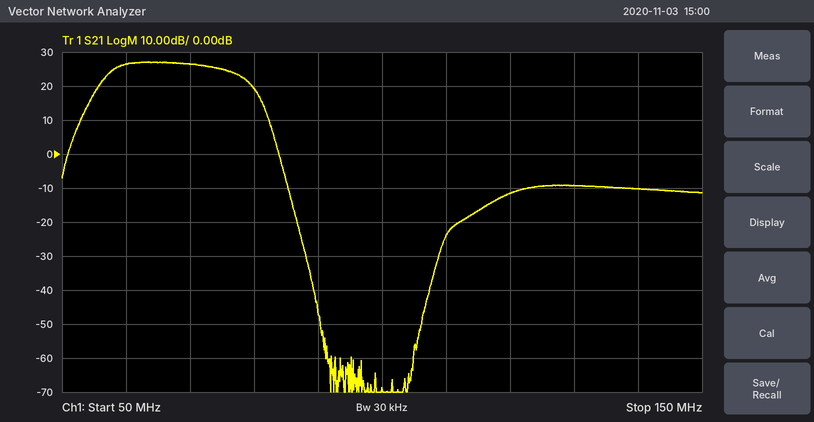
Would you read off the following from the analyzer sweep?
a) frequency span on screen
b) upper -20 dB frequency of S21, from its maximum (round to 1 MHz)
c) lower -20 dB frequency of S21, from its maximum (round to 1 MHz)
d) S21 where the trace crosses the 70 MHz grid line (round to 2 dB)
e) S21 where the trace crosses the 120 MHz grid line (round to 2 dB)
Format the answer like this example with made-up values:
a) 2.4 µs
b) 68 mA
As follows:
a) 100 MHz
b) 83 MHz
c) 52 MHz
d) 26 dB
e) -12 dB
